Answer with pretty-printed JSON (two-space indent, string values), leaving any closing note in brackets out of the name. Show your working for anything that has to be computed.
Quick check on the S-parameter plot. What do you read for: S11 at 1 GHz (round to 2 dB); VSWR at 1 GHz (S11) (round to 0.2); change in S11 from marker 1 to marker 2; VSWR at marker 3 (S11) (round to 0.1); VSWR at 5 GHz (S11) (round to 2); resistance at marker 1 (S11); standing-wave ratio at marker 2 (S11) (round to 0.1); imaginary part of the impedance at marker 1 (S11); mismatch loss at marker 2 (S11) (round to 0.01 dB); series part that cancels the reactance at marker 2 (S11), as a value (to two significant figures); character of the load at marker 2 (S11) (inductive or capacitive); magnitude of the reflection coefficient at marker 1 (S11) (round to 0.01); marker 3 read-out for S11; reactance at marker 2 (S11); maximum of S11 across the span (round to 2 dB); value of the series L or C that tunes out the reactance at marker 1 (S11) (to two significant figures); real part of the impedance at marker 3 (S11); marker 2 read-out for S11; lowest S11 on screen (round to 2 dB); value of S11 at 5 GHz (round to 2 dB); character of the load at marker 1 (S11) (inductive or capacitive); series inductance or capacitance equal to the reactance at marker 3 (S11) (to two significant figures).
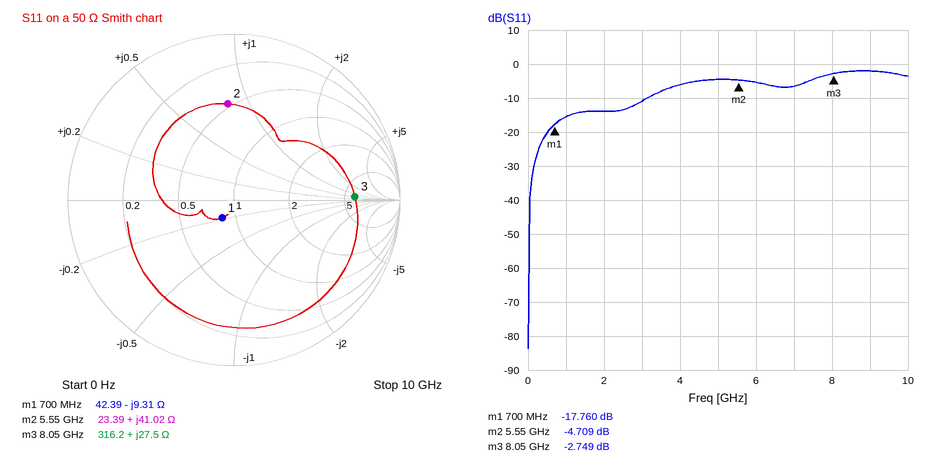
{
  "S11 at 1 GHz": "-16 dB",
  "VSWR at 1 GHz (S11)": "|Γ| = 10^(-16/20) = 0.1585; VSWR = (1 + 0.1585)/(1 − 0.1585) ≈ 1.4",
  "change in S11 from marker 1 to marker 2": "-4.709 − (-17.76) = 13.051 dB",
  "VSWR at marker 3 (S11)": "(1 + 0.7287)/(1 − 0.7287) ≈ 6.4",
  "VSWR at 5 GHz (S11)": "|Γ| = 10^(-4/20) = 0.6310; VSWR = (1 + 0.6310)/(1 − 0.6310) ≈ 4",
  "resistance at marker 1": "42.39 Ω",
  "standing-wave ratio at marker 2 (S11)": "3.8",
  "imaginary part of the impedance at marker 1": "-9.31 Ω",
  "mismatch loss at marker 2 (S11)": "−10 log10(1 − 10^(-4.709/10)) ≈ 1.79 dB",
  "series part that cancels the reactance at marker 2 (S11), as a value": "C = 1/(2π × 5.55 GHz × 41.02 Ω) ≈ 699 fF, so 700 fF to two significant figures",
  "character of the load at marker 2 (S11)": "inductive",
  "magnitude of the reflection coefficient at marker 1 (S11)": "10^(-17.76/20) ≈ 0.13",
  "marker 3 read-out for S11": "-2.749 dB",
  "reactance at marker 2": "+41.02 Ω",
  "maximum of S11 across the span": "-2 dB",
  "value of the series L or C that tunes out the reactance at marker 1 (S11)": "L = 9.31 Ω/(2π × 700 MHz) ≈ 2.1 nH",
  "real part of the impedance at marker 3": "316.2 Ω",
  "marker 2 read-out for S11": "-4.709 dB",
  "lowest S11 on screen": "-84 dB",
  "value of S11 at 5 GHz": "-4 dB",
  "character of the load at marker 1 (S11)": "capacitive",
  "series inductance or capacitance equal to the reactance at marker 3 (S11)": "L = 27.5 Ω/(2π × 8.05 GHz) ≈ 544 pH, so 540 pH to two significant figures"
}
